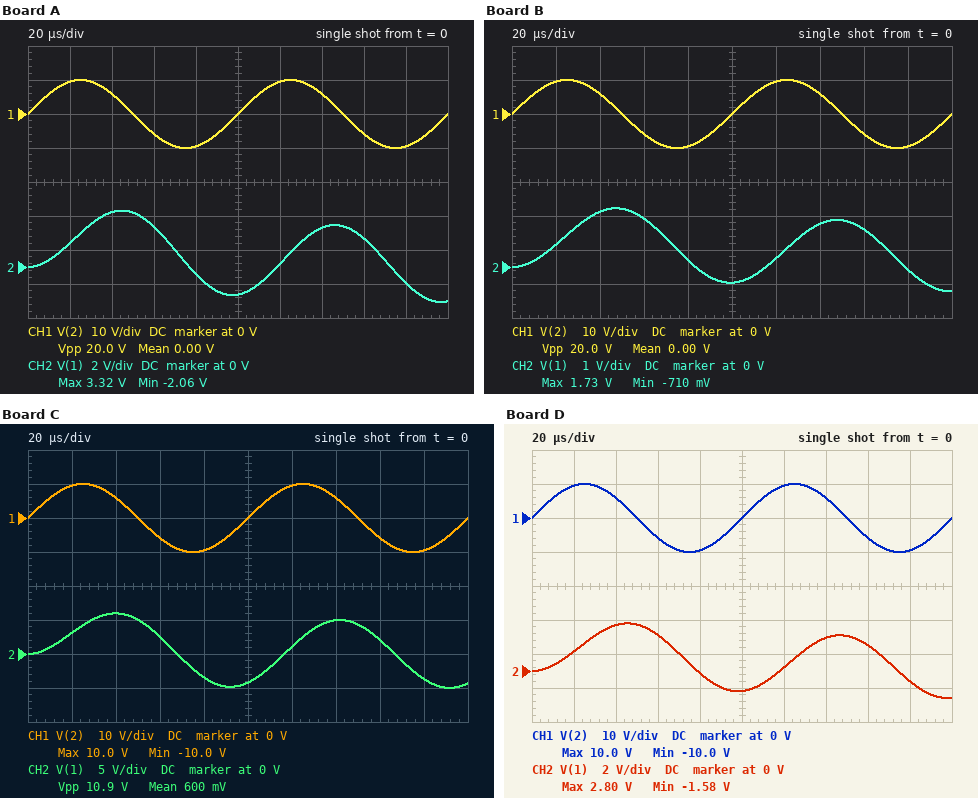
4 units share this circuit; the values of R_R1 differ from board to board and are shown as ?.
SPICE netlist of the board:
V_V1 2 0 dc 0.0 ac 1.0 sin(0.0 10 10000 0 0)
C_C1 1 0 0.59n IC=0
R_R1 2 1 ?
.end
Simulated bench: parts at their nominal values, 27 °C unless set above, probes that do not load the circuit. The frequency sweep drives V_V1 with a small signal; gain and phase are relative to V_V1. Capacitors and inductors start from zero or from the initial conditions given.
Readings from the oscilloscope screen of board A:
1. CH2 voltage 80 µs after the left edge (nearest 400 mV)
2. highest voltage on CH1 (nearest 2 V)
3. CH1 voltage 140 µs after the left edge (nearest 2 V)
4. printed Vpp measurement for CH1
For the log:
-400 mV
10 V
6 V
20.0 V
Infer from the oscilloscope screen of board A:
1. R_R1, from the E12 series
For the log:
120 kΩ
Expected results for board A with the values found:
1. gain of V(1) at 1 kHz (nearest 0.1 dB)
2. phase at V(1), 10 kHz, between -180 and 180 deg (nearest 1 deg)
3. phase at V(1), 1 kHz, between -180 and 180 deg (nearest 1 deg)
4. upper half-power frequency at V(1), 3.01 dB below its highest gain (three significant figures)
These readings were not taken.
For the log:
-0.8 dB
-77 deg
-24 deg
2.25 kHz
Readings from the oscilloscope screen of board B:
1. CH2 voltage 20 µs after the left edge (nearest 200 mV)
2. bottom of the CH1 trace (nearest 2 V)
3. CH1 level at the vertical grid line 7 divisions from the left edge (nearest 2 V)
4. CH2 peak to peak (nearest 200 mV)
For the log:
600 mV
-10 V
6 V
2.4 V
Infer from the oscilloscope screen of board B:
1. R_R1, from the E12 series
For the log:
270 kΩ
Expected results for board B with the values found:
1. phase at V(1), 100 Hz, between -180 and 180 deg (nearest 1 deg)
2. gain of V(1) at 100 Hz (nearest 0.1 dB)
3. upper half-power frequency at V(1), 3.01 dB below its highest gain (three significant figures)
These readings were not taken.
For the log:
-6 deg
0 dB
999 Hz
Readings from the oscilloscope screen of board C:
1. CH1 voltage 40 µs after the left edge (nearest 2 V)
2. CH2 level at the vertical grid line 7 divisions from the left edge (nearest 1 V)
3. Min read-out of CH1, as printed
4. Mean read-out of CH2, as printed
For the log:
6 V
5 V
-10.0 V
600 mV
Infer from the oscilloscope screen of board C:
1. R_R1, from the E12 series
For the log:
47 kΩ
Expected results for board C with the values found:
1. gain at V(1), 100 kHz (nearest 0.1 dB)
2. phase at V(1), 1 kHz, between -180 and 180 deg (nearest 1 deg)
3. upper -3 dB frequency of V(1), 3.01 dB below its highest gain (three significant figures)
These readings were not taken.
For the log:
-24.8 dB
-10 deg
5.74 kHz
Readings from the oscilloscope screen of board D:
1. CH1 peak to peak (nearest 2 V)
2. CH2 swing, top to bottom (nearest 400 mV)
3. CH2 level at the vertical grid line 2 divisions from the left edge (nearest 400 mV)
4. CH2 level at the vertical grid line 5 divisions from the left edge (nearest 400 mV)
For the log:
20 V
4.4 V
2.8 V
-1.2 V
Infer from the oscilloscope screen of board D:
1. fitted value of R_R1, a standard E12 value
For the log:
150 kΩ
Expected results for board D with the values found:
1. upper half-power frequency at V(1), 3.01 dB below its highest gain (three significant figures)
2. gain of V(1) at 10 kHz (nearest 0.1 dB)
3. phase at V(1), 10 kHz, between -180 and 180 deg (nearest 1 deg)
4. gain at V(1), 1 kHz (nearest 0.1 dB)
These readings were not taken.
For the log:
1.80 kHz
-15.0 dB
-80 deg
-1.2 dB
